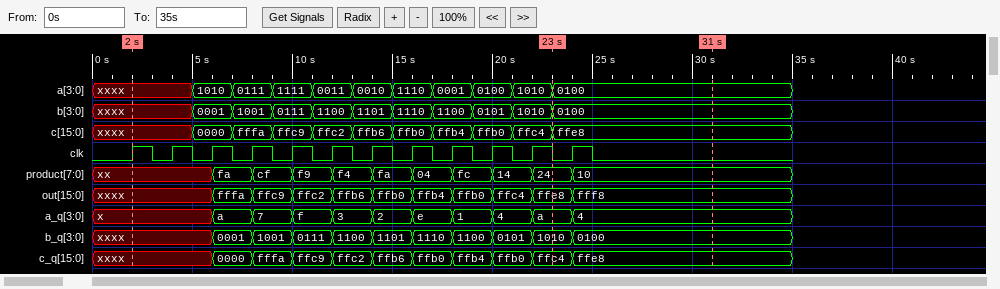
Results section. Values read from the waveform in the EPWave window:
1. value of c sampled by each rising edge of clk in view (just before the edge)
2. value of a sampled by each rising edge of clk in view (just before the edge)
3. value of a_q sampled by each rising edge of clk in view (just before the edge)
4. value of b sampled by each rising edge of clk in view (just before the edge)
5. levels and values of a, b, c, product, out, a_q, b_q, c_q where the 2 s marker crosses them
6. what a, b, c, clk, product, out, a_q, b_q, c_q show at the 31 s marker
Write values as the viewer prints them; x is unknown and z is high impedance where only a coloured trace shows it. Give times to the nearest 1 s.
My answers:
xxxx, xxxx, 0000, fffa, ffc9, ffc2, ffb6, ffb0, ffb4, ffb0, ffc4, ffe8
xxxx, xxxx, 1010, 0111, 1111, 0011, 0010, 1110, 0001, 0100, 1010, 0100
x, x, x, a, 7, f, 3, 2, e, 1, 4, a
xxxx, xxxx, 0001, 1001, 0111, 1100, 1101, 1110, 1100, 0101, 1010, 0100
a=xxxx, b=xxxx, c=xxxx, product=xx, out=xxxx, a_q=x, b_q=xxxx, c_q=xxxx
a=0100, b=0100, c=ffe8, clk=0, product=10, out=fff8, a_q=4, b_q=0100, c_q=ffe8
